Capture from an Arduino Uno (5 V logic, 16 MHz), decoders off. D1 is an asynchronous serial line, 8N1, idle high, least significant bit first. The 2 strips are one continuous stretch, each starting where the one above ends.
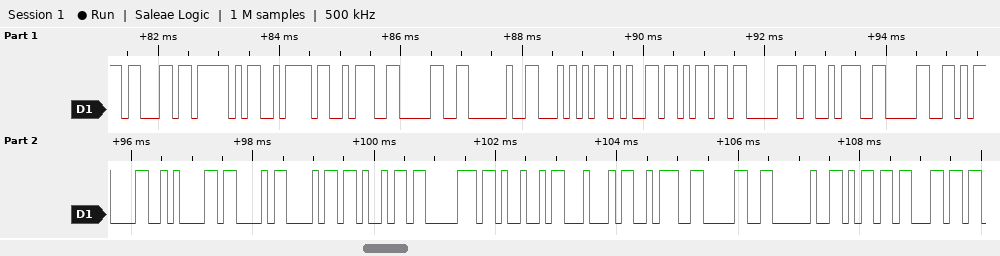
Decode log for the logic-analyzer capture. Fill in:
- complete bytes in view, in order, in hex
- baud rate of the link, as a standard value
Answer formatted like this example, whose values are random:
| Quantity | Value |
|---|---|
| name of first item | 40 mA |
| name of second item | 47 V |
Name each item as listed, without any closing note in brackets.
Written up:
| Quantity | Value |
|---|---|
| complete bytes in view, in order, in hex | 63 5F 7A 3A 30 20 54 65 6D 70 3A 30 0D 0A 43 68 69 70 49 44 3A 30 20 6D 6C |
| baud rate of the link, as a standard value | 9600 baud |
